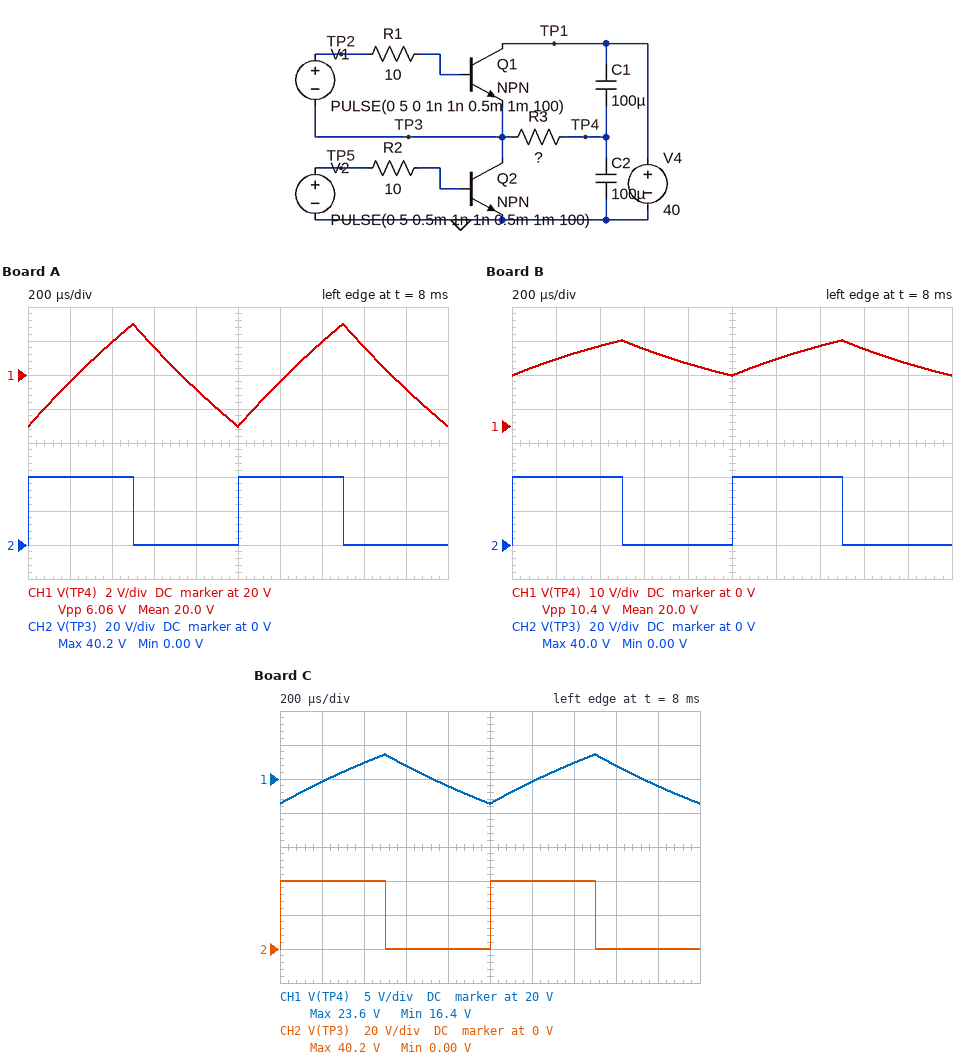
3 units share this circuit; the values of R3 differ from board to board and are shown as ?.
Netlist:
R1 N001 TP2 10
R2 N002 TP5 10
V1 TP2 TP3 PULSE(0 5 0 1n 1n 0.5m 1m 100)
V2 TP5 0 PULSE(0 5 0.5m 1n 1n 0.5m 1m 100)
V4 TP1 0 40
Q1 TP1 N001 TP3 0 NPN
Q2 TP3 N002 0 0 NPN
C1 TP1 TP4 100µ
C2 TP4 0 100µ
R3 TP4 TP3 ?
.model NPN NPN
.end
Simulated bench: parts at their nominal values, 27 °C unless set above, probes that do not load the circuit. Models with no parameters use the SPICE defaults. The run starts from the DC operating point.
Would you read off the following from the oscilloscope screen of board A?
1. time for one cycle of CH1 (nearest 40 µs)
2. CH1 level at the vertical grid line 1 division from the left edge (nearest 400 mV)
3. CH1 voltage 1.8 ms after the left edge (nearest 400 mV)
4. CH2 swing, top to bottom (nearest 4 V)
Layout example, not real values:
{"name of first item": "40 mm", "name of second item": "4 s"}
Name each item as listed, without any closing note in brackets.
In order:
{"time for one cycle of CH1": "1.00 ms", "CH1 level at the vertical grid line 1 division from the left edge": "19.6 V", "CH1 voltage 1.8 ms after the left edge": "19.2 V", "CH2 swing, top to bottom": "40 V"}
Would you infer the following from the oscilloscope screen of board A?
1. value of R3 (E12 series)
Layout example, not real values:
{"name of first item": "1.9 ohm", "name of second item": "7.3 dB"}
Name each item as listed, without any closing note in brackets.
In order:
{"value of R3": "8.2 Ω"}
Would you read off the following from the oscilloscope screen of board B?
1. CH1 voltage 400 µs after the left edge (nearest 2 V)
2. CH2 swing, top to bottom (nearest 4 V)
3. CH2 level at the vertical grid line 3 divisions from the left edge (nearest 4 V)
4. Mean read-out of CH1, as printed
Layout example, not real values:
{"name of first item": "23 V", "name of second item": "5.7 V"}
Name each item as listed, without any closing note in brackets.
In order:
{"CH1 voltage 400 µs after the left edge": "24 V", "CH2 swing, top to bottom": "40 V", "CH2 level at the vertical grid line 3 divisions from the left edge": "0 V", "Mean read-out of CH1, as printed": "20.0 V"}
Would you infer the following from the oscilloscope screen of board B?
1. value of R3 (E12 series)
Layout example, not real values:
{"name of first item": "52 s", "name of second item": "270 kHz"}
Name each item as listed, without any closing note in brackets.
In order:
{"value of R3": "4.7 Ω"}
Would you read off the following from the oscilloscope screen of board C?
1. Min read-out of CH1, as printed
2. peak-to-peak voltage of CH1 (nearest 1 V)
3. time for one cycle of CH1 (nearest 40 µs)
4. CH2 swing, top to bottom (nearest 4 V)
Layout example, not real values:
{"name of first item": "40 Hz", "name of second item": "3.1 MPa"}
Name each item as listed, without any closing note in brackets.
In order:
{"Min read-out of CH1, as printed": "16.4 V", "peak-to-peak voltage of CH1": "7 V", "time for one cycle of CH1": "1.00 ms", "CH2 swing, top to bottom": "40 V"}
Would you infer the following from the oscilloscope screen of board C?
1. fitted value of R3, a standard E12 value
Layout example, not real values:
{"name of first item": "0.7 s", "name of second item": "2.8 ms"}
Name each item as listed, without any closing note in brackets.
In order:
{"fitted value of R3, a standard E12 value": "6.8 Ω"}
